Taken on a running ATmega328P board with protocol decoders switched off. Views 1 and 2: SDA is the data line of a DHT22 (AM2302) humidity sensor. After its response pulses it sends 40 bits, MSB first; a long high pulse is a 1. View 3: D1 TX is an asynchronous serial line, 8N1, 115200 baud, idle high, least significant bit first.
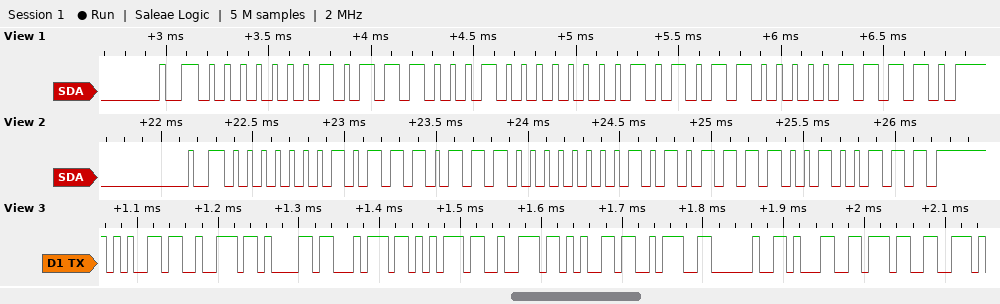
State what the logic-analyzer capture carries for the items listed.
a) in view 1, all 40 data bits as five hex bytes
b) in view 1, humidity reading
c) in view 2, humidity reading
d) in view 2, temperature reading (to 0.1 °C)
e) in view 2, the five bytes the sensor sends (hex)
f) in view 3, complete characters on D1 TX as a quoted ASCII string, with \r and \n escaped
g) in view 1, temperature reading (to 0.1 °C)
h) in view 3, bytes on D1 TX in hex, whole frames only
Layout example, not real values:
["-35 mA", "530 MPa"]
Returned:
["01 71 00 AC 1E", "36.9 %", "37.5 %", "17.5 °C", "01 77 00 AF 27", "\"erature: 17\"", "17.2 °C", "65 72 61 74 75 72 65 3A 20 31 37"]
